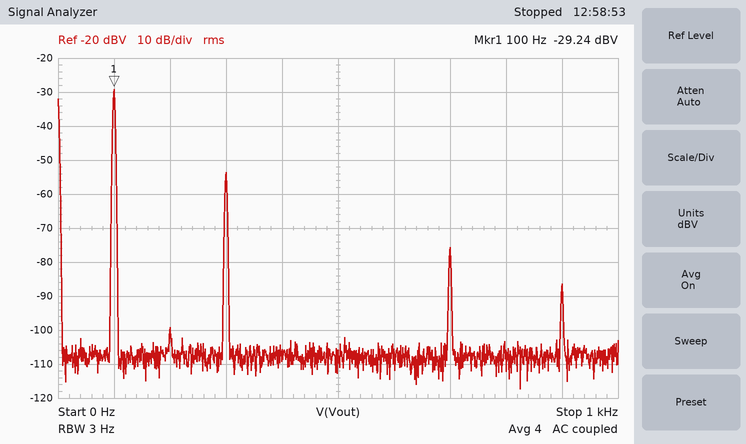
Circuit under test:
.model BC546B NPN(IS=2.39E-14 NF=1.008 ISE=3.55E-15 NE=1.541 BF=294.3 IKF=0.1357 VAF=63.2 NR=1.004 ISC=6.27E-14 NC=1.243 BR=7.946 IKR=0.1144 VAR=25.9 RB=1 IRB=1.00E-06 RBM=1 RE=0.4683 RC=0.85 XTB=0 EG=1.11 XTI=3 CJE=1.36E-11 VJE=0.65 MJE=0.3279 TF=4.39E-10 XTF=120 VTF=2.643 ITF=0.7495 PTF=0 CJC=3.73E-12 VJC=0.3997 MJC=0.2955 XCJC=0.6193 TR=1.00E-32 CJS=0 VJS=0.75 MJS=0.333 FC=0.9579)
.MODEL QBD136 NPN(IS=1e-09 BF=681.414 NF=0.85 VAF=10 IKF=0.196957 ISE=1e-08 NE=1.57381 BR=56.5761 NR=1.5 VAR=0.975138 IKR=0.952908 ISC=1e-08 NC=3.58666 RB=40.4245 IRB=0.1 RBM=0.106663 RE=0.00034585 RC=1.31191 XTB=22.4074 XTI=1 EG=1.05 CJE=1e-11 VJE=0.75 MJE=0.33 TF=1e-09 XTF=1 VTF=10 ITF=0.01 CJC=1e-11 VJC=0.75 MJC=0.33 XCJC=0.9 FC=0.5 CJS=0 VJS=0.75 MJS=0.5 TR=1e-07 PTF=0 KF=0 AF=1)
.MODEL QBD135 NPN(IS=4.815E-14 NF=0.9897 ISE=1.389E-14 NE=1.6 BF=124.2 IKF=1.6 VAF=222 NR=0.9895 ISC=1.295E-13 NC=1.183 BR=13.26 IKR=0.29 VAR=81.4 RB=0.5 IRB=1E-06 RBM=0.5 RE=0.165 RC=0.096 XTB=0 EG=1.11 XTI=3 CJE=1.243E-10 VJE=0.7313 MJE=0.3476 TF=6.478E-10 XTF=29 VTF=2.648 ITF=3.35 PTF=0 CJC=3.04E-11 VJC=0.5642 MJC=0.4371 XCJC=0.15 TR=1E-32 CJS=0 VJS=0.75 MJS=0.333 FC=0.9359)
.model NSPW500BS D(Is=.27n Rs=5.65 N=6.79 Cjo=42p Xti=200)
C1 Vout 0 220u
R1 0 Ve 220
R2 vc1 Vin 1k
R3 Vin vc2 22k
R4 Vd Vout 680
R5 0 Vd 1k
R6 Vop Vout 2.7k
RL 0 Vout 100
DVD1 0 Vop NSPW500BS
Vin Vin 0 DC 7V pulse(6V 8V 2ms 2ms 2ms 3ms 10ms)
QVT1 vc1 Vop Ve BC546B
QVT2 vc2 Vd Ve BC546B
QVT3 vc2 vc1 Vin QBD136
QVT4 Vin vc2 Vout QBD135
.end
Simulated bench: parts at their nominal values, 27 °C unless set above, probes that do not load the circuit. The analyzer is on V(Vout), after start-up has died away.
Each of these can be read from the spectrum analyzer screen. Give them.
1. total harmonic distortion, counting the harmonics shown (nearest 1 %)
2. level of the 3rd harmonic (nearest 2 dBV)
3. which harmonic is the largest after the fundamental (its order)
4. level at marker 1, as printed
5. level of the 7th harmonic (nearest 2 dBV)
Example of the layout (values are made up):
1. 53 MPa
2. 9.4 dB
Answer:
1. 6 %
2. -54 dBV
3. 3
4. -29.24 dBV
5. -76 dBV
